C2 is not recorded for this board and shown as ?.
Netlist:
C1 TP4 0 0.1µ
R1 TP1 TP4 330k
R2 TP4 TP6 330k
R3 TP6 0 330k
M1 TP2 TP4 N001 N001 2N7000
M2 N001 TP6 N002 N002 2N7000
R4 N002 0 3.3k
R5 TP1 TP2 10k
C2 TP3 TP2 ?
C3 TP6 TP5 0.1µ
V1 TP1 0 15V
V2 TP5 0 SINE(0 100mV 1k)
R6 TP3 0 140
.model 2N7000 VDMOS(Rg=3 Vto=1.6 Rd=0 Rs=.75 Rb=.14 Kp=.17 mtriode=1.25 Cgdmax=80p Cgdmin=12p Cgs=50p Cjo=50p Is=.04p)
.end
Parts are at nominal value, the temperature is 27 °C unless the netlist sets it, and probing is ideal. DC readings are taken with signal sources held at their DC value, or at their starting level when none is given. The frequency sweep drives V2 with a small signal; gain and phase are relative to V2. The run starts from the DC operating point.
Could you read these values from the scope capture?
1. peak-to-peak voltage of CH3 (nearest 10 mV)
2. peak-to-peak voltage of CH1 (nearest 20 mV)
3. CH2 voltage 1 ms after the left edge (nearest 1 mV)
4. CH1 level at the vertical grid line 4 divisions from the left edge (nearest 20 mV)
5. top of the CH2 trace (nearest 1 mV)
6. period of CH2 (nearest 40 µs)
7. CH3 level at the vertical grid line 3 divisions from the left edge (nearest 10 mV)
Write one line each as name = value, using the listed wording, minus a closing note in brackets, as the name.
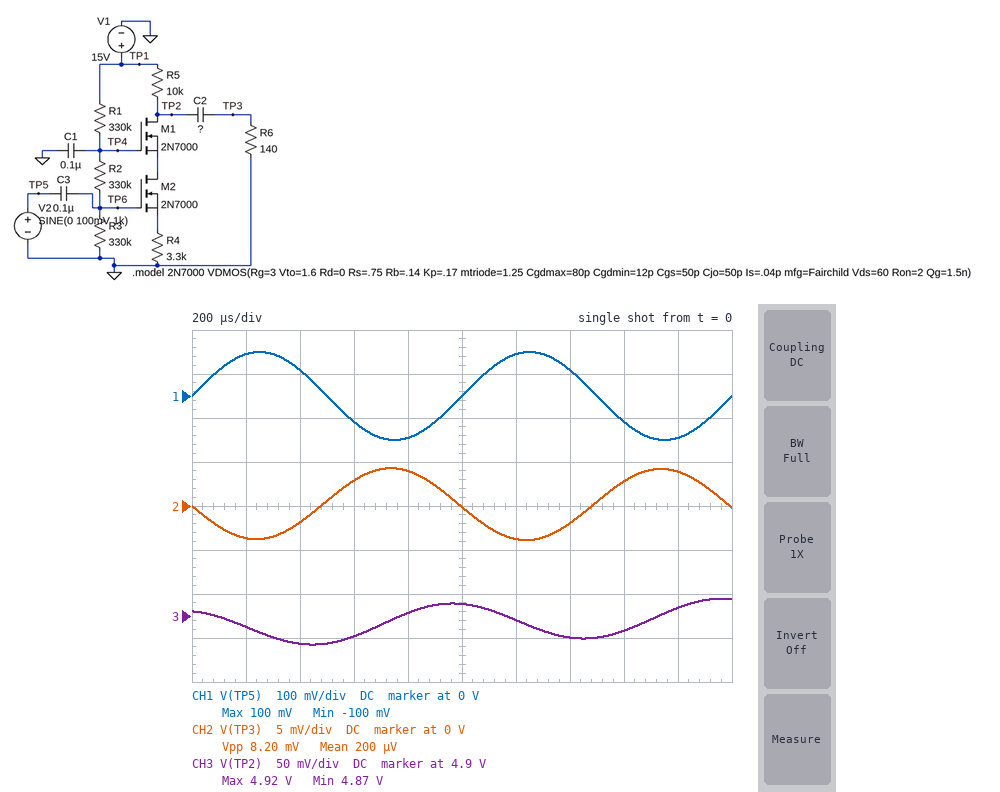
peak-to-peak voltage of CH3 = 50 mV
peak-to-peak voltage of CH1 = 200 mV
CH2 voltage 1 ms after the left edge = 0 V
CH1 level at the vertical grid line 4 divisions from the left edge = -100 mV
top of the CH2 trace = 4 mV
period of CH2 = 1.00 ms
CH3 level at the vertical grid line 3 divisions from the left edge = 4.88 V
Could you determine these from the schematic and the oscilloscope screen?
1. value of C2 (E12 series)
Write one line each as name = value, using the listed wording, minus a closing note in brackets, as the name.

value of C2 = 220 nF
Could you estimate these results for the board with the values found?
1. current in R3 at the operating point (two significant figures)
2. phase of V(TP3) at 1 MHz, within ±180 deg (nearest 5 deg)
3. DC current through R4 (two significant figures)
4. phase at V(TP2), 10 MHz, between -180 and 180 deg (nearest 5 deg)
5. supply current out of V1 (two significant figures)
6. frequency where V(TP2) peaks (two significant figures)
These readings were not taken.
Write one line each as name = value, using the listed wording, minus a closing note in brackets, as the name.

current in R3 at the operating point = 15 µA
phase of V(TP3) at 1 MHz, within ±180 deg = 120 deg
DC current through R4 = 1.0 mA
phase at V(TP2), 10 MHz, between -180 and 180 deg = 40 deg
supply current out of V1 = 1.0 mA
frequency where V(TP2) peaks = 28 Hz
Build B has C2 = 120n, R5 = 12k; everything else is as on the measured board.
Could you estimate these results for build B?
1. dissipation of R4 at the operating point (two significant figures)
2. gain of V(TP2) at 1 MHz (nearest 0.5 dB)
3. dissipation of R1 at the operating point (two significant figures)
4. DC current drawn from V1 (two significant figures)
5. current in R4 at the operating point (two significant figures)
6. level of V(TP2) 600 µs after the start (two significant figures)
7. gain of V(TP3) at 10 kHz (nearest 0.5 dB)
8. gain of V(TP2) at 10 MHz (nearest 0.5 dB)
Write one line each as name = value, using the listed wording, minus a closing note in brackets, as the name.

dissipation of R4 at the operating point = 3.2 mW
gain of V(TP2) at 1 MHz = -20.0 dB
dissipation of R1 at the operating point = 76 µW
DC current drawn from V1 = 990 µA
current in R4 at the operating point = 980 µA
level of V(TP2) 600 µs after the start = 3.3 V
gain of V(TP3) at 10 kHz = -45.5 dB
gain of V(TP2) at 10 MHz = -7.5 dB
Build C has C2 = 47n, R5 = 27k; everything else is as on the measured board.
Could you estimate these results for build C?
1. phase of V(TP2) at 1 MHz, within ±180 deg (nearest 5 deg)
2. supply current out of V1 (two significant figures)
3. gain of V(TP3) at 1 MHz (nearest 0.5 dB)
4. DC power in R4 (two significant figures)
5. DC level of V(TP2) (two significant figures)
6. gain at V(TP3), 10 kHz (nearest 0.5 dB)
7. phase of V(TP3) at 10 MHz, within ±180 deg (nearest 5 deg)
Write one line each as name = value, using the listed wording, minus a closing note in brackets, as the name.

phase of V(TP2) at 1 MHz, within ±180 deg = 75 deg
supply current out of V1 = 510 µA
gain of V(TP3) at 1 MHz = -19.5 dB
DC power in R4 = 810 µW
DC level of V(TP2) = 1.6 V
gain at V(TP3), 10 kHz = -59.5 dB
phase of V(TP3) at 10 MHz, within ±180 deg = 25 deg
